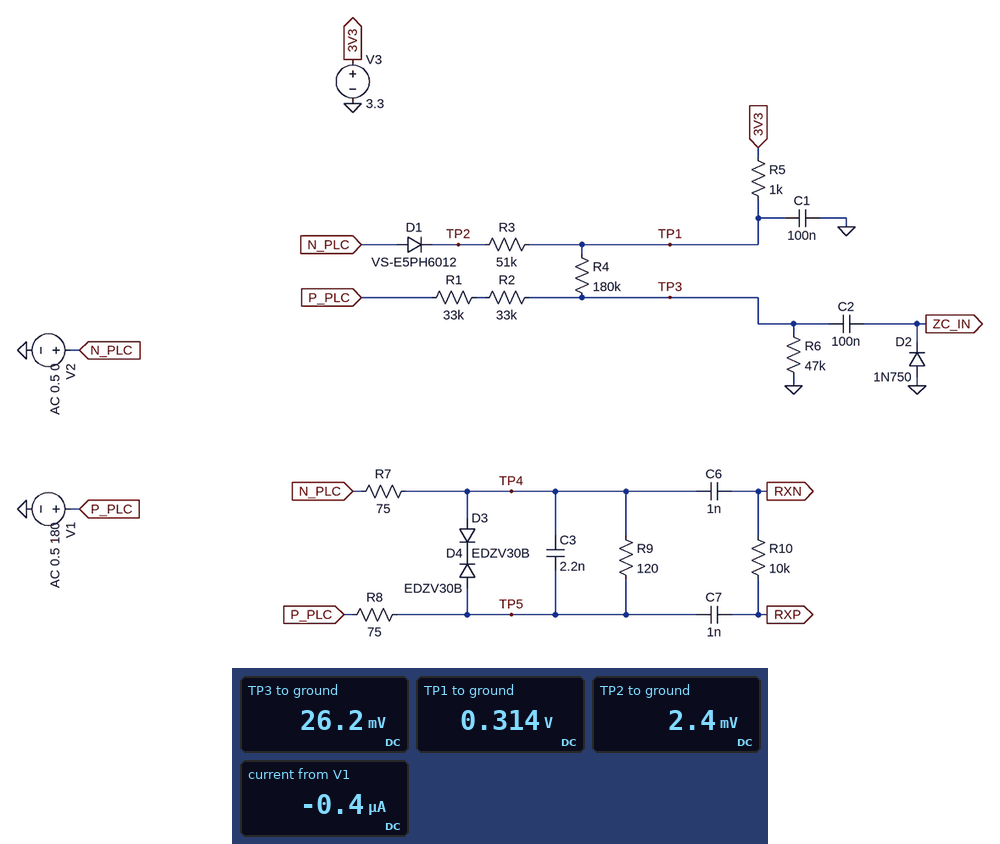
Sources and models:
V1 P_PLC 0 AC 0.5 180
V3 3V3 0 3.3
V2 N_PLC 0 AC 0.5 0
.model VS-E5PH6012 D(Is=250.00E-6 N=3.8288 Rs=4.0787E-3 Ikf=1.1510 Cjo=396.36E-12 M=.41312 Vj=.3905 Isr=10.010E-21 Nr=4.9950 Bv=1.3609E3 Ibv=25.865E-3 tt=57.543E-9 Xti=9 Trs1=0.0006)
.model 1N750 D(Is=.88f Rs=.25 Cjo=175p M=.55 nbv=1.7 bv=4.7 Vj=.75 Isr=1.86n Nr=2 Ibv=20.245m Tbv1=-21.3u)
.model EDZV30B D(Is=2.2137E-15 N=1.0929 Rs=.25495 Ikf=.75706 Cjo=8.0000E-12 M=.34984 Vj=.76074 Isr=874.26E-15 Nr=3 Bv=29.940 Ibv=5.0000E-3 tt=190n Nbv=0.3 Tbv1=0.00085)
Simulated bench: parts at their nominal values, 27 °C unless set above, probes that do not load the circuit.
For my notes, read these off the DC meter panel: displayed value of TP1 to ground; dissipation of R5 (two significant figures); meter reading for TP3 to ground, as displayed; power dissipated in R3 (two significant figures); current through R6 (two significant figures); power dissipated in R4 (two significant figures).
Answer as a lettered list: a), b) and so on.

a) 0.314 V
b) 8.9 mW
c) 26.2 mV
d) 1.9 µW
e) 560 nA
f) 460 nW
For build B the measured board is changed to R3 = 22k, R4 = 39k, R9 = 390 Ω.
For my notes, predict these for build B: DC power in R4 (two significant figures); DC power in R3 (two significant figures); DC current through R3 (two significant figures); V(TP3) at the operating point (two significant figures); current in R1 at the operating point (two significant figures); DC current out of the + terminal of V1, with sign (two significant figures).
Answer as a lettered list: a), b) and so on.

a) 1.2 µW
b) 4.3 µW
c) 14 µA
d) 96 mV
e) 1.5 µA
f) -1.5 µA
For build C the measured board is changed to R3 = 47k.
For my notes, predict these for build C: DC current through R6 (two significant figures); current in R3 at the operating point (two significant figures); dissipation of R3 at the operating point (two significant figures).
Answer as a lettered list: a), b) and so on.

a) 560 nA
b) 6.6 µA
c) 2.1 µW
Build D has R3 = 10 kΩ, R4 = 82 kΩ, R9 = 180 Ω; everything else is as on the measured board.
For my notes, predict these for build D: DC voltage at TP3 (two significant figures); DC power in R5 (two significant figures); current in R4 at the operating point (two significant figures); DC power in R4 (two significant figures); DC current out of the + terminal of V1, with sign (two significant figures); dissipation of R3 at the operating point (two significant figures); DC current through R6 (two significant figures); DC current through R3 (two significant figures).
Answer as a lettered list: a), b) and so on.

a) 53 mV
b) 8.9 mW
c) 3.2 µA
d) 820 nW
e) -800 nA
f) 9.0 µW
g) 1.1 µA
h) 30 µA
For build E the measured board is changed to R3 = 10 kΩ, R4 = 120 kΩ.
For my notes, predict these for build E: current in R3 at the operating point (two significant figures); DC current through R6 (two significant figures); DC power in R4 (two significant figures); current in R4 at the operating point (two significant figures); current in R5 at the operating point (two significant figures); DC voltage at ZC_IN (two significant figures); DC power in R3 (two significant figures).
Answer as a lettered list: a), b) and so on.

a) 30 µA
b) 810 nA
c) 630 nW
d) 2.3 µA
e) 3.0 mA
f) 38 mV
g) 9.0 µW
